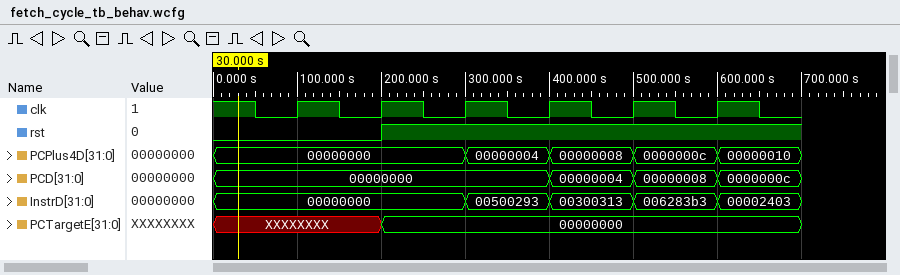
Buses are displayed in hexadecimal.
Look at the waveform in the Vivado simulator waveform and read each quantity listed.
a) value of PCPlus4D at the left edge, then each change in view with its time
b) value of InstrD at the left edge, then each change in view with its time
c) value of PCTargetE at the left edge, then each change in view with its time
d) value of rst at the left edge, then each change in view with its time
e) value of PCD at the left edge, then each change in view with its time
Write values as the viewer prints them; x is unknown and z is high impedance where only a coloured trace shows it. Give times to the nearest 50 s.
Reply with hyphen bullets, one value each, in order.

- 00000000, 00000004 at 300 s, 00000008 at 400 s, 0000000c at 500 s, 00000010 at 600 s
- 00000000, 00500293 at 300 s, 00300313 at 400 s, 006283b3 at 500 s, 00002403 at 600 s
- XXXXXXXX, 00000000 at 200 s
- 0, 1 at 200 s
- 00000000, 00000004 at 400 s, 00000008 at 500 s, 0000000c at 600 s
